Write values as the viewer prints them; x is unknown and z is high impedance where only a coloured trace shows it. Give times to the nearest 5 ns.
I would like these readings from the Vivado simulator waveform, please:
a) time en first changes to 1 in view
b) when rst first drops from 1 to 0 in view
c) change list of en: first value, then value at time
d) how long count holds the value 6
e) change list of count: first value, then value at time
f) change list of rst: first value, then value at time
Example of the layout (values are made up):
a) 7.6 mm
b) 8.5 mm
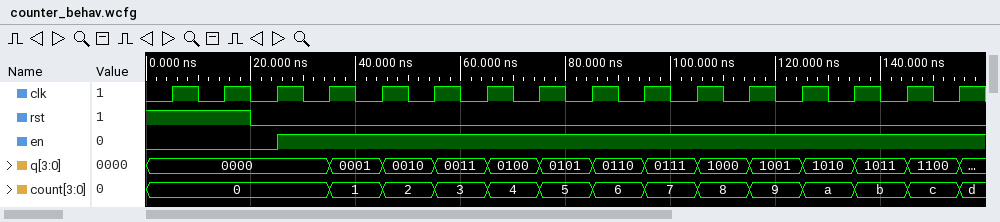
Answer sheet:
a) 25 ns
b) 20 ns
c) 0, 1 at 25 ns
d) 10 ns
e) 0, 1 at 35 ns, 2 at 45 ns, 3 at 55 ns, 4 at 65 ns, 5 at 75 ns, 6 at 85 ns, 7 at 95 ns, 8 at 105 ns, 9 at 115 ns, a at 125 ns, b at 135 ns, c at 145 ns, d at 155 ns
f) 1, 0 at 20 ns
